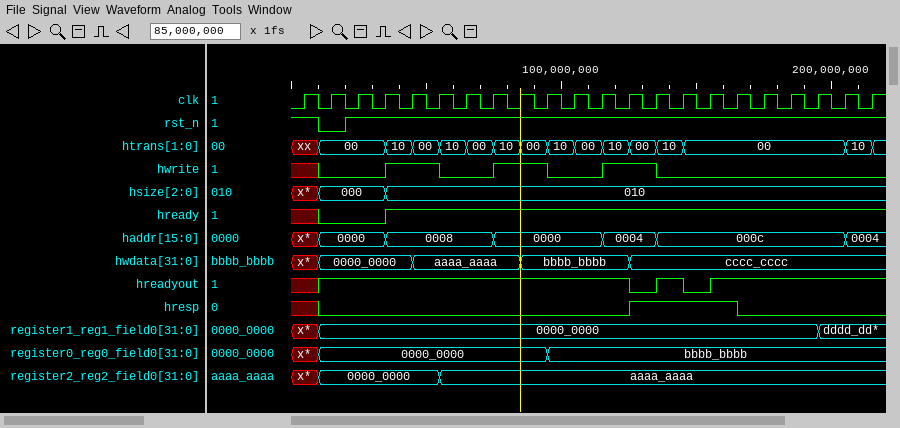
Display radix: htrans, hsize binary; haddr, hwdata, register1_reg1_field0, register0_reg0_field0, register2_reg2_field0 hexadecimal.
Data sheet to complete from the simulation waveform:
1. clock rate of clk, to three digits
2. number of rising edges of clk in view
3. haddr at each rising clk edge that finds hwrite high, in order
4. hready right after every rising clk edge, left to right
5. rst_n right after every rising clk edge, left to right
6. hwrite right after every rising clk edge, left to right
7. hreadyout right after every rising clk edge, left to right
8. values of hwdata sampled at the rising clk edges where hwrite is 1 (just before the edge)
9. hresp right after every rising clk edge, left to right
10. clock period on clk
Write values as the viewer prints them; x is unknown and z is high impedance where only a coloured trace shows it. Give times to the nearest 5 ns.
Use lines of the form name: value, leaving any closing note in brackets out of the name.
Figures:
clock rate of clk, to three digits: 100 MHz
number of rising edges of clk in view: 22
haddr at each rising clk edge that finds hwrite high, in order: 0008, 0008, 0000, 0000, 0004, 0004
hready right after every rising clk edge, left to right: x 0 0 1 1 1 1 1 1 1 1 1 1 1 1 1 1 1 1 1 1 1
rst_n right after every rising clk edge, left to right: 1 0 1 1 1 1 1 1 1 1 1 1 1 1 1 1 1 1 1 1 1 1
hwrite right after every rising clk edge, left to right: x 0 0 1 1 0 0 1 1 0 0 1 1 0 0 0 0 0 0 0 0 0
hreadyout right after every rising clk edge, left to right: x 1 1 1 1 1 1 1 1 1 1 1 0 1 0 1 1 1 1 1 1 1
values of hwdata sampled at the rising clk edges where hwrite is 1: 0000_0000, aaaa_aaaa, aaaa_aaaa, bbbb_bbbb, bbbb_bbbb, cccc_cccc
hresp right after every rising clk edge, left to right: x 0 0 0 0 0 0 0 0 0 0 0 1 1 1 1 0 0 0 0 0 0
clock period on clk: 10 ns
